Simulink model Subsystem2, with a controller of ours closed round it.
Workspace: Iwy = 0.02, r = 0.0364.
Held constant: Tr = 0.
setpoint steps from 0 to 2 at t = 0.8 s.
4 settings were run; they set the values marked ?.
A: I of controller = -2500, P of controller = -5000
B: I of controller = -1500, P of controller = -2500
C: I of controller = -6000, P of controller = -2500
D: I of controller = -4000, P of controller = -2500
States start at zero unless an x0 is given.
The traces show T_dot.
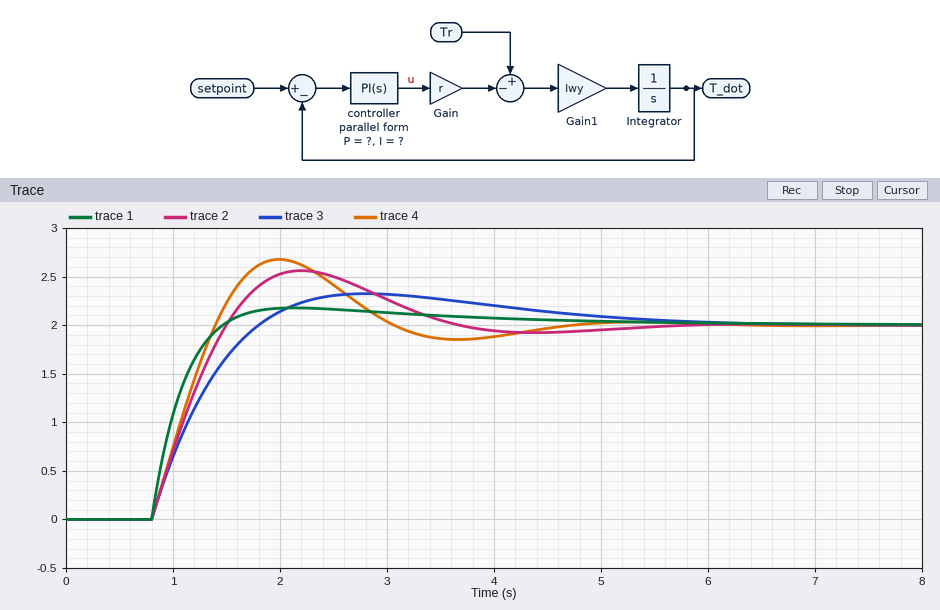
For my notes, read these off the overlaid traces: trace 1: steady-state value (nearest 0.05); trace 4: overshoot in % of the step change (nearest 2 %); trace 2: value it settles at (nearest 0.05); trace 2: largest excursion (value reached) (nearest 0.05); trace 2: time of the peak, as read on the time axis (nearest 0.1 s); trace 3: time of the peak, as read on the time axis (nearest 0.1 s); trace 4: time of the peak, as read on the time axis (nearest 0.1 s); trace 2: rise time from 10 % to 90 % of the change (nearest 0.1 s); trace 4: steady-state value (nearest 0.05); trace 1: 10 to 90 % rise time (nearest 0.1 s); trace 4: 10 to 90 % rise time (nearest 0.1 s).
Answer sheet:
2.00
34 %
2.00
2.55
2.2 s
2.8 s
2.0 s
0.5 s
2.00
0.5 s
0.5 s
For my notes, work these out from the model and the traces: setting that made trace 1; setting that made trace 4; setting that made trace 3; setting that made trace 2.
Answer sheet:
A
C
B
D
